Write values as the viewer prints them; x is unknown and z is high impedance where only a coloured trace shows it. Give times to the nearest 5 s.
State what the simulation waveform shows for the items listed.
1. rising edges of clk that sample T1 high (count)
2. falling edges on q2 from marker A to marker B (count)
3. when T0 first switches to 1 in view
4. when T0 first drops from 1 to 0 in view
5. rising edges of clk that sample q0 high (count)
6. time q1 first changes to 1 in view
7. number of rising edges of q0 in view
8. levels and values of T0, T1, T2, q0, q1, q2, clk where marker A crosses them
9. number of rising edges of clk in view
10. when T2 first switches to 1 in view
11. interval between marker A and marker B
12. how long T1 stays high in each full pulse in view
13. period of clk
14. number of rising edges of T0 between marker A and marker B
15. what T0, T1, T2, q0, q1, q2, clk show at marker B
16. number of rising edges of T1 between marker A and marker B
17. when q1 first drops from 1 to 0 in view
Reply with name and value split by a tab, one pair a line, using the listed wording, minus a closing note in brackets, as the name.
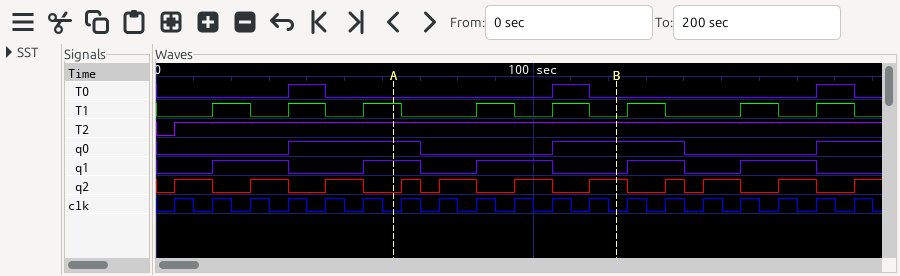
rising edges of clk that sample T1 high	8
falling edges on q2 from marker A to marker B	3
when T0 first switches to 1 in view	35 s
when T0 first drops from 1 to 0 in view	45 s
rising edges of clk that sample q0 high	7
time q1 first changes to 1 in view	15 s
number of rising edges of q0 in view	3
levels and values of T0, T1, T2, q0, q1, q2, clk where marker A crosses them	T0=0, T1=1, T2=1, q0=1, q1=1, q2=0, clk=0
number of rising edges of clk in view	19
when T2 first switches to 1 in view	5 s
interval between marker A and marker B	60 s
how long T1 stays high in each full pulse in view	10 s, 10 s, 10 s, 10 s, 10 s, 10 s, 10 s, 10 s
period of clk	10 s
number of rising edges of T0 between marker A and marker B	1
what T0, T1, T2, q0, q1, q2, clk show at marker B	T0=0, T1=0, T2=1, q0=1, q1=0, q2=1, clk=0
number of rising edges of T1 between marker A and marker B	2
when q1 first drops from 1 to 0 in view	35 s
